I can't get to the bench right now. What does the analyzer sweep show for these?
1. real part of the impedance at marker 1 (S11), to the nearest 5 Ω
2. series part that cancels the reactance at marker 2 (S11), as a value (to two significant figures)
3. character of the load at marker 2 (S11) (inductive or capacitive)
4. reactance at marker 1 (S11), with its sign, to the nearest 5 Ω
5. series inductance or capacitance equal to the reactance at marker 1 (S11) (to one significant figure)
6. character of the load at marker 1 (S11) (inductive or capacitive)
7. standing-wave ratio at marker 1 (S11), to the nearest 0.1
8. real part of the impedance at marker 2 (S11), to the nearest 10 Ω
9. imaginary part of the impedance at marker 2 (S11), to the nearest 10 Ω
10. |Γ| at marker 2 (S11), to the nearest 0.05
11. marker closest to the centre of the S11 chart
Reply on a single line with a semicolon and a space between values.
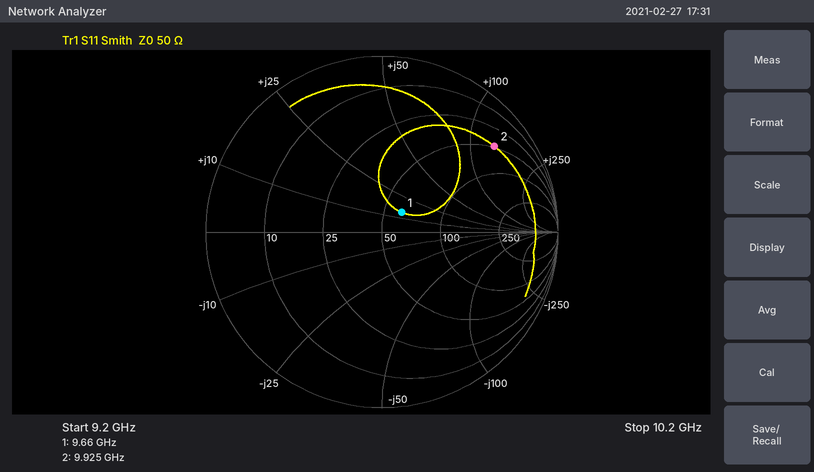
60 Ω; 120 fF; inductive; +15 Ω; 200 pH; inductive; 1.4; 50 Ω; +130 Ω; 0.80; marker 1
